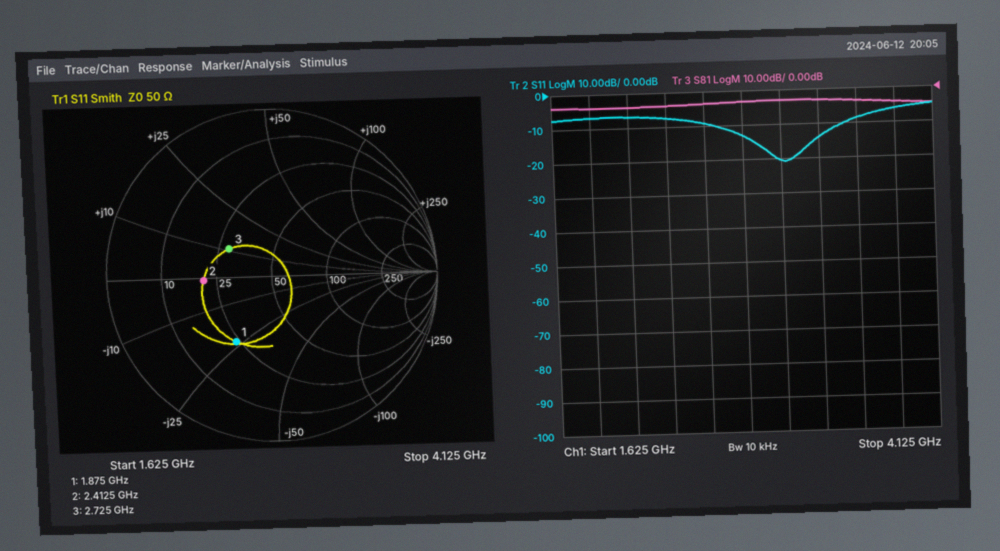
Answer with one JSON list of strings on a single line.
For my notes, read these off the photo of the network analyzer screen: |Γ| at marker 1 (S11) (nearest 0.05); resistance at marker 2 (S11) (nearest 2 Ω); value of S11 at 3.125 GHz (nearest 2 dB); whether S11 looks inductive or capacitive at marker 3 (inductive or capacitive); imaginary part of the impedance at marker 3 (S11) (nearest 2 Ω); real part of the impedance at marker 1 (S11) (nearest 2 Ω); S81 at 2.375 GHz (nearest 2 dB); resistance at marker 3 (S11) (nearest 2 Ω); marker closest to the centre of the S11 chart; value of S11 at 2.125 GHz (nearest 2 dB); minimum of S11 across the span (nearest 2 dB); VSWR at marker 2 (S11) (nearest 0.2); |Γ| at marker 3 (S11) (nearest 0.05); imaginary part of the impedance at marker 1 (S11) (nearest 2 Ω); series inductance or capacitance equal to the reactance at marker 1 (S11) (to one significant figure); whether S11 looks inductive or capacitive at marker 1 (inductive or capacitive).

["0.45", "20 Ω", "-20 dB", "inductive", "+10 Ω", "24 Ω", "-4 dB", "28 Ω", "marker 3", "-6 dB", "-20 dB", "2.4", "0.30", "-24 Ω", "4 pF", "capacitive"]
